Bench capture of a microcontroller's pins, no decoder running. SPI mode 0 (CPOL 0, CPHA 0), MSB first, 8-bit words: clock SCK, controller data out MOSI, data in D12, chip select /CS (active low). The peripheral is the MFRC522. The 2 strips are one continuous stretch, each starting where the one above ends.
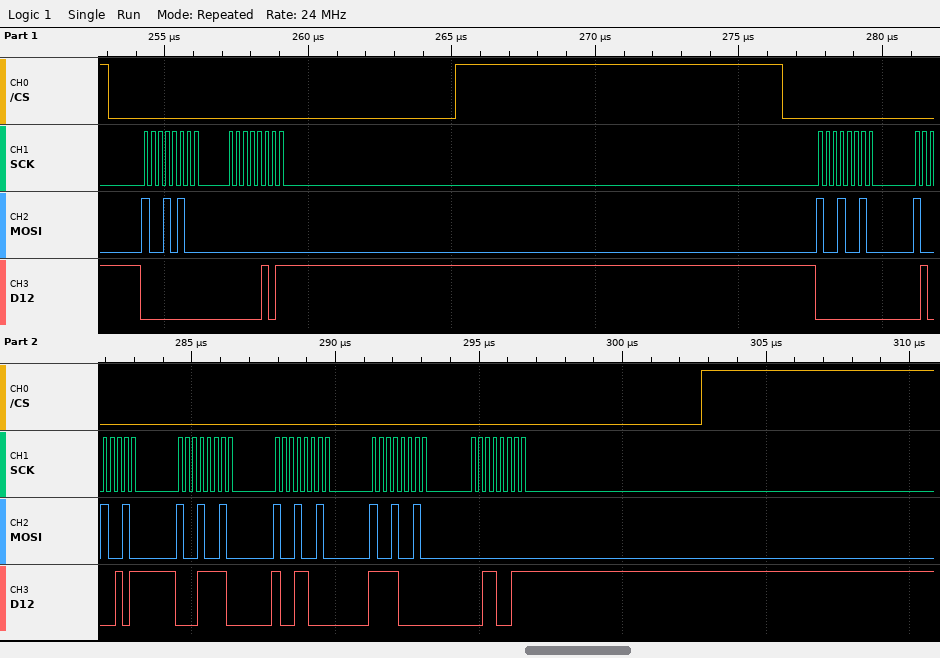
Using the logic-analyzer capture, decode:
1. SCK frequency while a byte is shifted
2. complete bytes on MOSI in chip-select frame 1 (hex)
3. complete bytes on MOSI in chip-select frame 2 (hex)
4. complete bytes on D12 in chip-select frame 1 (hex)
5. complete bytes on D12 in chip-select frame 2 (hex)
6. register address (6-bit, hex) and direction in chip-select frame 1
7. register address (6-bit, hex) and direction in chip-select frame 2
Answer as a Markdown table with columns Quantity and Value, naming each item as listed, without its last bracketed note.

| Quantity | Value |
|---|---|
| SCK frequency while a byte is shifted | 4 MHz |
| complete bytes on MOSI in chip-select frame 1 | 94 00 |
| complete bytes on MOSI in chip-select frame 2 | 92 92 92 92 92 00 |
| complete bytes on D12 in chip-select frame 1 | 00 05 |
| complete bytes on D12 in chip-select frame 2 | 00 45 1E 98 F0 33 |
| register address (6-bit, hex) and direction in chip-select frame 1 | 0x0A read |
| register address (6-bit, hex) and direction in chip-select frame 2 | 0x09 read |
